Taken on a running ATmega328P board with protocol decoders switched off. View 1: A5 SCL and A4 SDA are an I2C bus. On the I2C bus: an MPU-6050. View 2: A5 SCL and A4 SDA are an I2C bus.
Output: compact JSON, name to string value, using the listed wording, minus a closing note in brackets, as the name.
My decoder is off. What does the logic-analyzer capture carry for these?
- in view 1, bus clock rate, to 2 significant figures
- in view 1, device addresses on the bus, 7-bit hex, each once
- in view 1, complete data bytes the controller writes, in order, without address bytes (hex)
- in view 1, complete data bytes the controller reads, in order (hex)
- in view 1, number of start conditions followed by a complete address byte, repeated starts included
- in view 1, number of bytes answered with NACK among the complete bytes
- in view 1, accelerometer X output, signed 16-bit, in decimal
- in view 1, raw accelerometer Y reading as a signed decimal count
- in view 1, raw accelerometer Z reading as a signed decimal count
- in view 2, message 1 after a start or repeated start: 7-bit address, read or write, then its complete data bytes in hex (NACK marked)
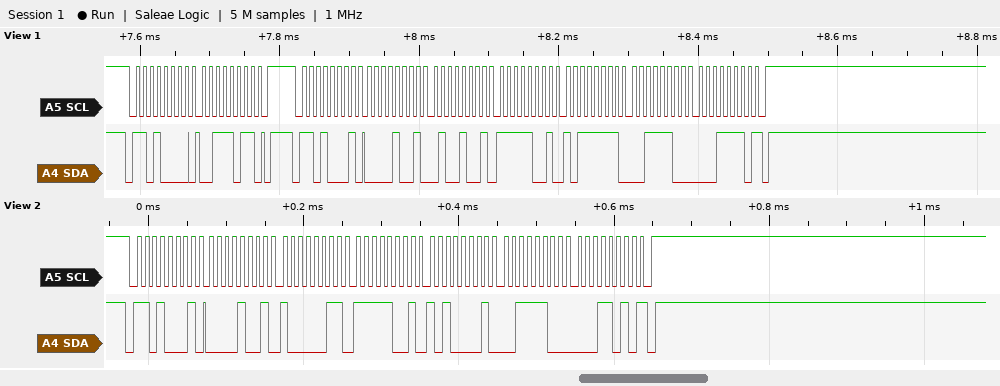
{"in view 1, bus clock rate, to 2 significant figures": "100 kHz", "in view 1, device addresses on the bus, 7-bit hex, each once": "0x68", "in view 1, complete data bytes the controller writes, in order, without address bytes": "3B", "in view 1, complete data bytes the controller reads, in order": "09 49 F9 BF 3C 1E", "in view 1, number of start conditions followed by a complete address byte, repeated starts included": "2", "in view 1, number of bytes answered with NACK among the complete bytes": "1", "in view 1, accelerometer X output, signed 16-bit, in decimal": "2377", "in view 1, raw accelerometer Y reading as a signed decimal count": "-1601", "in view 1, raw accelerometer Z reading as a signed decimal count": "15390", "in view 2, message 1 after a start or repeated start: 7-bit address, read or write, then its complete data bytes in hex": "0x68 read: 09 83 F9 A1 3C 1A NACK"}
